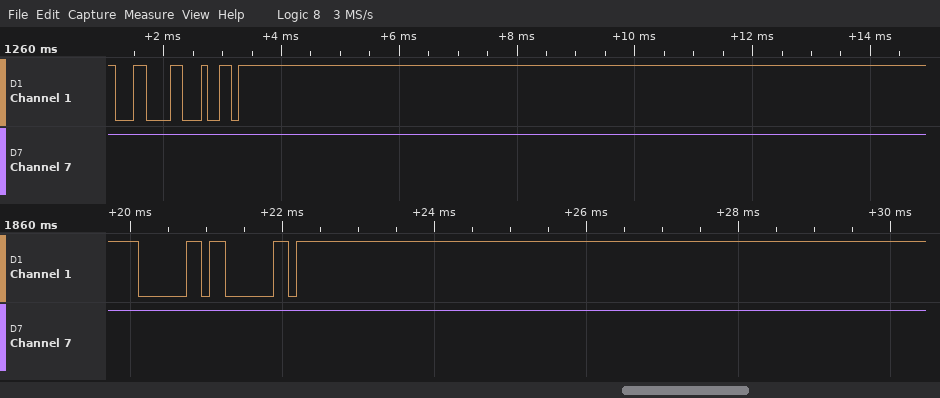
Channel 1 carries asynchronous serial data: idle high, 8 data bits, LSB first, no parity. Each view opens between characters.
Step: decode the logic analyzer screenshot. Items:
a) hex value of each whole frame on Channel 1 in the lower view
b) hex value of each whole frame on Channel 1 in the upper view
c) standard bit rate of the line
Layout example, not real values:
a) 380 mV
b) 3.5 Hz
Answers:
a) 60, 60
b) 0C, 64
c) 9600 baud
